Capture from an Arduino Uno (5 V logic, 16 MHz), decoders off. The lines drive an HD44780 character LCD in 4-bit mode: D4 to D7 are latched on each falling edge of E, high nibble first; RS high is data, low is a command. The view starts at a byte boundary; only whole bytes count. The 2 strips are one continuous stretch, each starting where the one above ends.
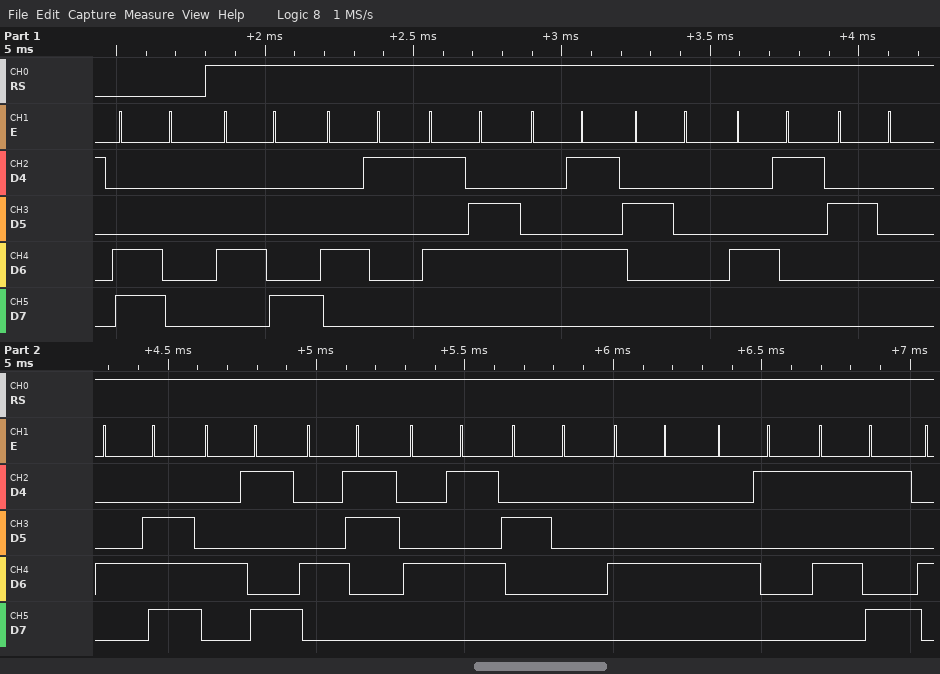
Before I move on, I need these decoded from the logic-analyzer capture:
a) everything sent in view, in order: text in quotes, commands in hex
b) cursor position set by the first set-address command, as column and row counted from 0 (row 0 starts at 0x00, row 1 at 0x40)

0xC0 "HAVE A NICE DAY"
column 0, row 1
